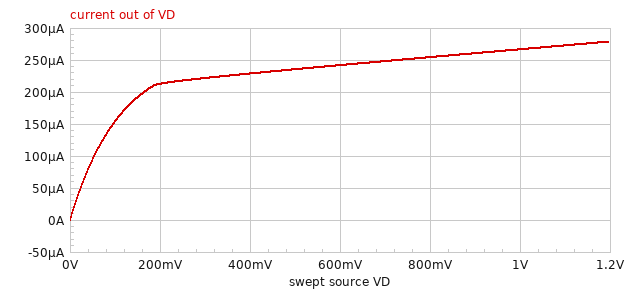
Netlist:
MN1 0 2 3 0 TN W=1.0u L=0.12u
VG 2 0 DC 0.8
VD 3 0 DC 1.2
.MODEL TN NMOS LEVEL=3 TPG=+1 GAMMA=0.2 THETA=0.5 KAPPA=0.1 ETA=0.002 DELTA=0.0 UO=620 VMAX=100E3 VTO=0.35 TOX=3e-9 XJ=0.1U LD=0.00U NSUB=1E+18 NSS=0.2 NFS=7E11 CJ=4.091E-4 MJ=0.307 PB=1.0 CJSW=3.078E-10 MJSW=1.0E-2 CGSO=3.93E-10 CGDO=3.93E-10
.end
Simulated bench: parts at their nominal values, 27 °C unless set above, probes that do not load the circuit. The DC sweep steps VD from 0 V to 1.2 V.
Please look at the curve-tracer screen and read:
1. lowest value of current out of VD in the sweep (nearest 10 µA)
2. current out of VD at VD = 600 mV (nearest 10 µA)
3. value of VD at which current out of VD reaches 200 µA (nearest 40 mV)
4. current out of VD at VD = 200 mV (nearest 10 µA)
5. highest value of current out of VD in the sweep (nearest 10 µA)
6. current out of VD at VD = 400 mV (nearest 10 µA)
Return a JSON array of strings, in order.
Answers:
["0 A", "240 µA", "160 mV", "210 µA", "280 µA", "230 µA"]
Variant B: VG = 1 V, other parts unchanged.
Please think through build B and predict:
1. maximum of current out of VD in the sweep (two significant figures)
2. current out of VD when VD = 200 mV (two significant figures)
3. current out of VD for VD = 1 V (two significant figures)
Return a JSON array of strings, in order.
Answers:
["390 µA", "310 µA", "380 µA"]
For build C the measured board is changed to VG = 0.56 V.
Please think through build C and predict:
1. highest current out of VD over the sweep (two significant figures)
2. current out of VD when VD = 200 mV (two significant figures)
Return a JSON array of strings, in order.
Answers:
["150 µA", "95 µA"]
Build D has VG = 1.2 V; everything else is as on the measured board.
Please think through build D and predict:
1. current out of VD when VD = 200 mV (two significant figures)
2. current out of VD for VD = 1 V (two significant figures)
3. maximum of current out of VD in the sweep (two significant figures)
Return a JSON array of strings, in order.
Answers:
["390 µA", "490 µA", "510 µA"]
